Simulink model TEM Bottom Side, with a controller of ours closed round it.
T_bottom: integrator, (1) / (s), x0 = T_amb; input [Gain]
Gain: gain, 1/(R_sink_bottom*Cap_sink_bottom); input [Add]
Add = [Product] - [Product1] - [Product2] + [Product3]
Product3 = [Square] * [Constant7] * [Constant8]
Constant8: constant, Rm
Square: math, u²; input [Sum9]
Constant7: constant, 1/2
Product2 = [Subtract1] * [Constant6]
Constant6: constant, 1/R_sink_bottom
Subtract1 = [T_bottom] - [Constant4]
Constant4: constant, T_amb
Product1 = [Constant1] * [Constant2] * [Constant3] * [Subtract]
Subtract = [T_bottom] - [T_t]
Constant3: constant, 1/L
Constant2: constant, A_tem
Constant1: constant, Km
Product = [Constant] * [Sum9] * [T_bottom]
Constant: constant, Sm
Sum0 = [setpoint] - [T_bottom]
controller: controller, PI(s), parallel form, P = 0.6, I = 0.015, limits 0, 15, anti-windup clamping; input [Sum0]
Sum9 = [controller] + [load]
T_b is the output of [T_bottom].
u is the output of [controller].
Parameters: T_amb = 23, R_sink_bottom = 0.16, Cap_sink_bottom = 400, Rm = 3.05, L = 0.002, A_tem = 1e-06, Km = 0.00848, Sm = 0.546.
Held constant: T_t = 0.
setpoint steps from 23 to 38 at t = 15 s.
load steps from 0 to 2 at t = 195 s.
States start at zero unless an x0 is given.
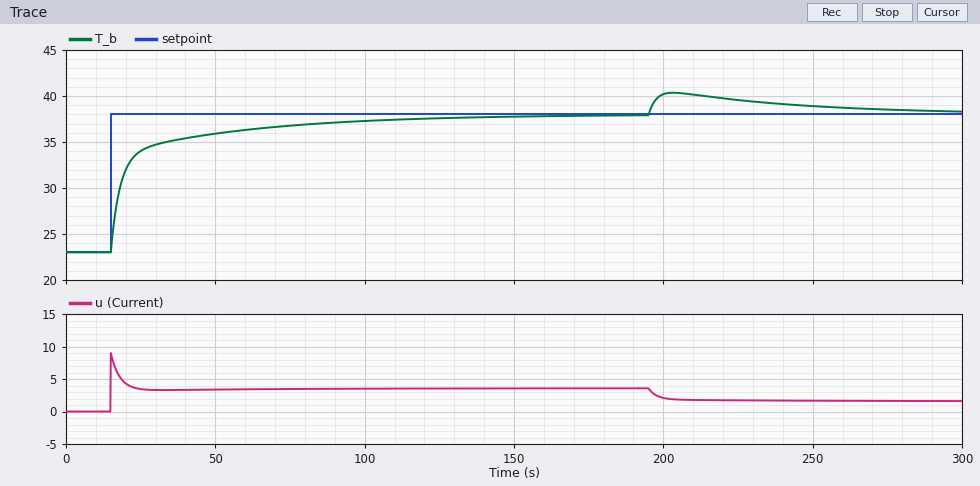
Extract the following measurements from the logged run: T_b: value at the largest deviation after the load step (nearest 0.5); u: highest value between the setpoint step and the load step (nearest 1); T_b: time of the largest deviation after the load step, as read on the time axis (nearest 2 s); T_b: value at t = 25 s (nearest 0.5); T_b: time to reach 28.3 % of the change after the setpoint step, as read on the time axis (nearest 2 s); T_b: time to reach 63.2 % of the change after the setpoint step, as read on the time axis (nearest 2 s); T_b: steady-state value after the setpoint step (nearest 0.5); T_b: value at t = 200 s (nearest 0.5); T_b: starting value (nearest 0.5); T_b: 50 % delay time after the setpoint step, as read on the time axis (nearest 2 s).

40.5
9
204 s
34.0
16 s
20 s
38.0
40.0
23.0
18 s
